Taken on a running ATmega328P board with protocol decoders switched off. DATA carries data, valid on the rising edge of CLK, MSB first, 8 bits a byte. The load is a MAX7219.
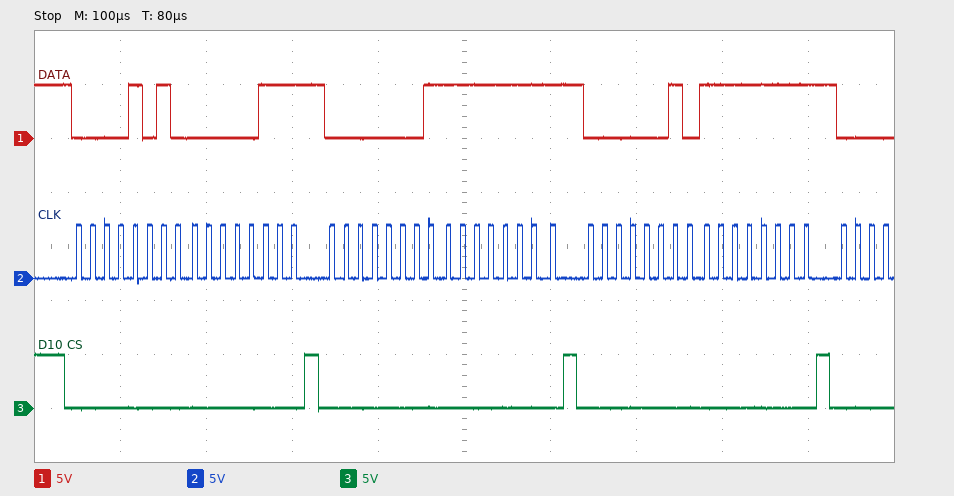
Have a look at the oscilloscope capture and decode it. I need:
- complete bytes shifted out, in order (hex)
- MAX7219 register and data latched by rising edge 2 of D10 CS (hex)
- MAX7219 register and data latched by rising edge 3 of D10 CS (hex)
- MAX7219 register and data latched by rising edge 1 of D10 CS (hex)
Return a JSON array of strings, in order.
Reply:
["0A 07 01 FF 02 FF", "register 0x1, data 0xFF", "register 0x2, data 0xFF", "register 0xA, data 0x07"]
